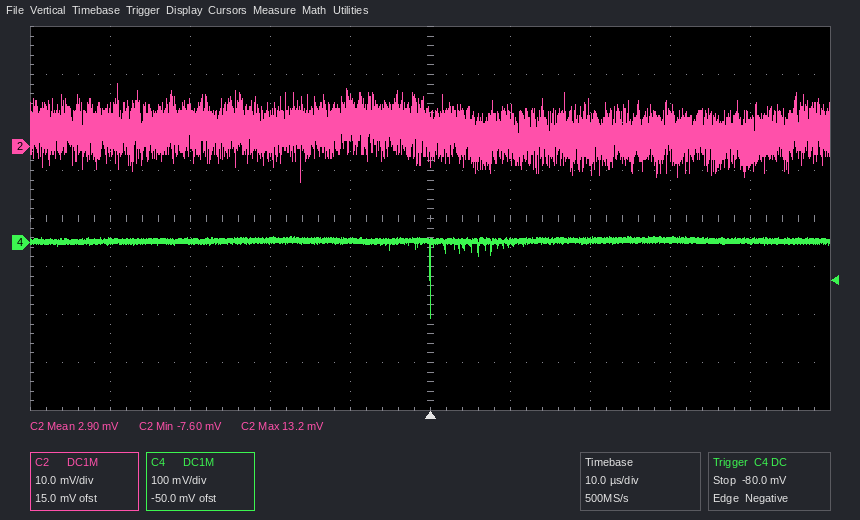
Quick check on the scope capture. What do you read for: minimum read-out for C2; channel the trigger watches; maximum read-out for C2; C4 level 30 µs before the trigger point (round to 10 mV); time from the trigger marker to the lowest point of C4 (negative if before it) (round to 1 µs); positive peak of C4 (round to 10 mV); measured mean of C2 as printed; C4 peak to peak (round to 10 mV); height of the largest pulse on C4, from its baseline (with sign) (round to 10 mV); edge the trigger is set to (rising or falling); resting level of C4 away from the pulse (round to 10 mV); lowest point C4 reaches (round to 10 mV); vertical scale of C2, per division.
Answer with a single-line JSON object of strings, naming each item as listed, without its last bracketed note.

{"minimum read-out for C2": "-7.60 mV", "channel the trigger watches": "C4", "maximum read-out for C2": "13.2 mV", "C4 level 30 µs before the trigger point": "0 mV", "time from the trigger marker to the lowest point of C4 (negative if before it)": "0 µs", "positive peak of C4": "10 mV", "measured mean of C2 as printed": "2.90 mV", "C4 peak to peak": "170 mV", "height of the largest pulse on C4, from its baseline (with sign)": "-160 mV", "edge the trigger is set to": "falling", "resting level of C4 away from the pulse": "0 mV", "lowest point C4 reaches": "-160 mV", "vertical scale of C2, per division": "10 mV"}
